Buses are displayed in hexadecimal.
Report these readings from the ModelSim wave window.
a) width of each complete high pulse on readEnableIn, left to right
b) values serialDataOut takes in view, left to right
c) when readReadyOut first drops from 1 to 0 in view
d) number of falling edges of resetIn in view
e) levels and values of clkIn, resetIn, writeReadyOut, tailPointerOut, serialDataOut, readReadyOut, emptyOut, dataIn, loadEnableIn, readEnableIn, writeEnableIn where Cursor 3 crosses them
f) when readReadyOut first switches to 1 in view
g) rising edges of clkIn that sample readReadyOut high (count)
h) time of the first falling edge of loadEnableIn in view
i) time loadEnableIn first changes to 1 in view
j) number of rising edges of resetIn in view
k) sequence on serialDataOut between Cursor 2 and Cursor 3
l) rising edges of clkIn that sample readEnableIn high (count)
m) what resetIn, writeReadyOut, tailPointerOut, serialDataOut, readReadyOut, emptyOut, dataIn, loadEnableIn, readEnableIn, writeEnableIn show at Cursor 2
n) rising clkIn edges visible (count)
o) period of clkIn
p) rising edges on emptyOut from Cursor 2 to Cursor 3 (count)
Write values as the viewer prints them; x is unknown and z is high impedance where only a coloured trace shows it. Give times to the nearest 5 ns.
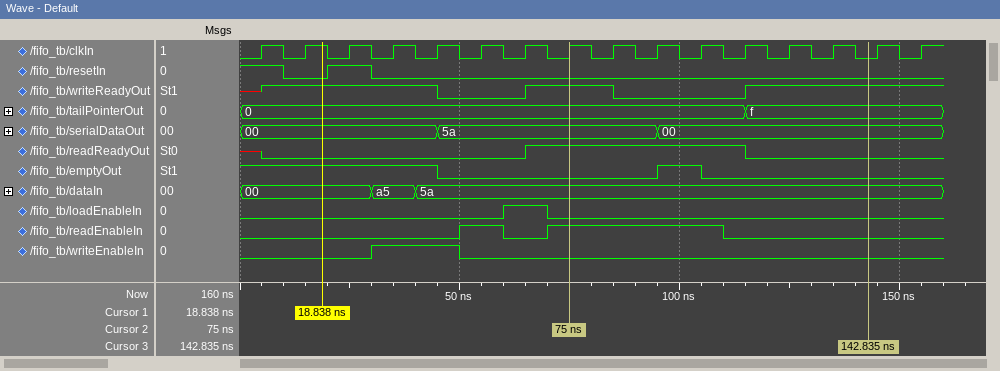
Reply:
10 ns, 40 ns
00, 5a, 00
115 ns
2
clkIn=0, resetIn=0, writeReadyOut=1, tailPointerOut=f, serialDataOut=00, readReadyOut=0, emptyOut=0, dataIn=5a, loadEnableIn=0, readEnableIn=0, writeEnableIn=0
65 ns
5
70 ns
60 ns
1
5a, 00
5
resetIn=0, writeReadyOut=1, tailPointerOut=0, serialDataOut=5a, readReadyOut=1, emptyOut=0, dataIn=5a, loadEnableIn=0, readEnableIn=1, writeEnableIn=0
16
10 ns
1
